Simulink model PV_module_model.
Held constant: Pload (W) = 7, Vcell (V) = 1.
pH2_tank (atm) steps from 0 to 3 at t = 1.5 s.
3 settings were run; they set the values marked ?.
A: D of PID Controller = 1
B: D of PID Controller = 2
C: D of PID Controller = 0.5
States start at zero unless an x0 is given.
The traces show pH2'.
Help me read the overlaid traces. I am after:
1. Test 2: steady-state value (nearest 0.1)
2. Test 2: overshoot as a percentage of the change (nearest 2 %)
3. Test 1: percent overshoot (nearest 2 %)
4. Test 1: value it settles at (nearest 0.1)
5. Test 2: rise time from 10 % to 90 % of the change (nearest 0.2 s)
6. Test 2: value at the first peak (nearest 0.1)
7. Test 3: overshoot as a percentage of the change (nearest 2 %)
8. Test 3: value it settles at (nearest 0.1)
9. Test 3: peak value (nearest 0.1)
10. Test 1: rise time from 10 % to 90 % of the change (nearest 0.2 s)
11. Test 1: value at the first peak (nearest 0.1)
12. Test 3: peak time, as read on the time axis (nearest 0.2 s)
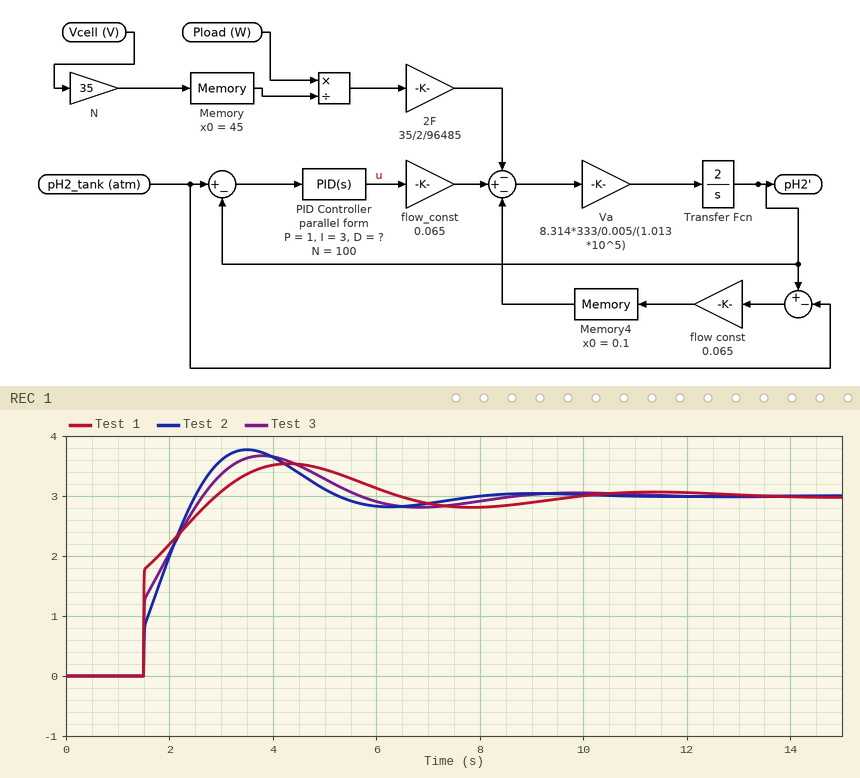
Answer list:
3.0
26 %
18 %
3.0
0.8 s
3.8
22 %
3.0
3.7
1.0 s
3.5
3.8 s
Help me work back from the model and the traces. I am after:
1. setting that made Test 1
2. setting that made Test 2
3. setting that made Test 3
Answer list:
B
C
A
